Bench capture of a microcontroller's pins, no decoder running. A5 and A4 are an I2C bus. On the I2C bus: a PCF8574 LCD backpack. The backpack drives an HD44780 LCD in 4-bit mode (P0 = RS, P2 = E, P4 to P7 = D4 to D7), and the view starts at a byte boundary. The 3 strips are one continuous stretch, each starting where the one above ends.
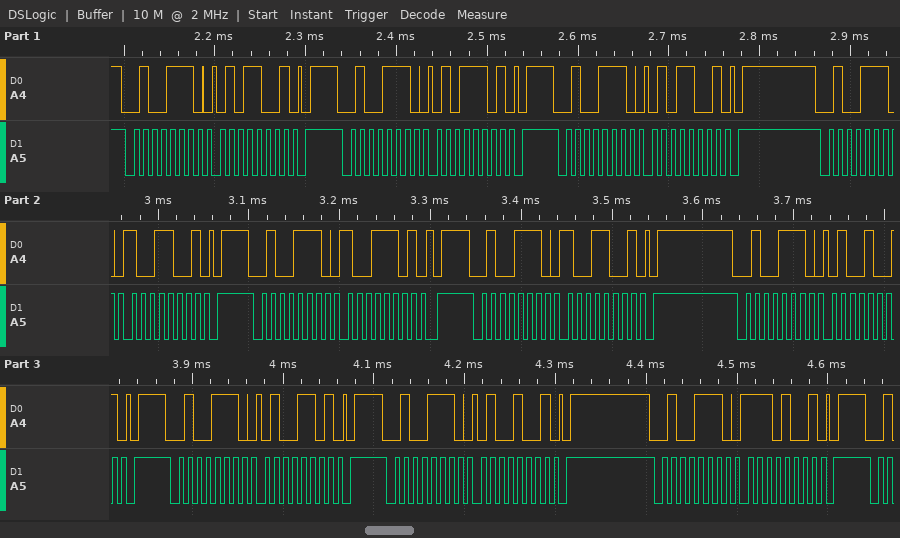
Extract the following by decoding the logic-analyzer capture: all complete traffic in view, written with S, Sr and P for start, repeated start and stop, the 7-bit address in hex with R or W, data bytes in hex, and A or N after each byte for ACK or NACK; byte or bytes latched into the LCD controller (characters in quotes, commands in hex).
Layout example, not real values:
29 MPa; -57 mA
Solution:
S 27W A 59 A P S 27W A 5D A P S 27W A 59 A P S 27W A 99 A P S 27W A 9D A P S 27W A 99 A P S 27W A 49 A P S 27W A 4D A P S 27W A 49 A P S 27W A E9 A P; 'Y'
